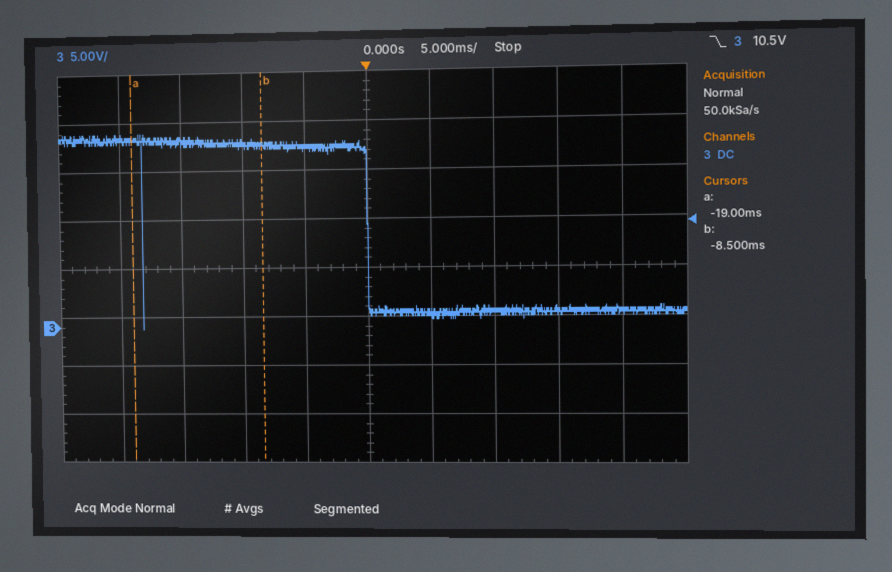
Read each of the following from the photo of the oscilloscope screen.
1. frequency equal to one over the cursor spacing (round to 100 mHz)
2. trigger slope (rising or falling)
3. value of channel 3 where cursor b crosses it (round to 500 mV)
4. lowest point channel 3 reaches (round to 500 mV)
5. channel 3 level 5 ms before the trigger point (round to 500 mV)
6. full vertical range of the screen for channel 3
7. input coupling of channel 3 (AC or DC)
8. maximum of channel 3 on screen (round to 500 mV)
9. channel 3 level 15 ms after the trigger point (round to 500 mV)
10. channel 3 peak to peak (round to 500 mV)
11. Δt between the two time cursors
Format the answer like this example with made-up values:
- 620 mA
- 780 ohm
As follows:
- 95.2 Hz
- falling
- 18.5 V
- 0.0 V
- 18.5 V
- 40 V
- DC
- 20.0 V
- 1.5 V
- 20.0 V
- 10.5 ms
